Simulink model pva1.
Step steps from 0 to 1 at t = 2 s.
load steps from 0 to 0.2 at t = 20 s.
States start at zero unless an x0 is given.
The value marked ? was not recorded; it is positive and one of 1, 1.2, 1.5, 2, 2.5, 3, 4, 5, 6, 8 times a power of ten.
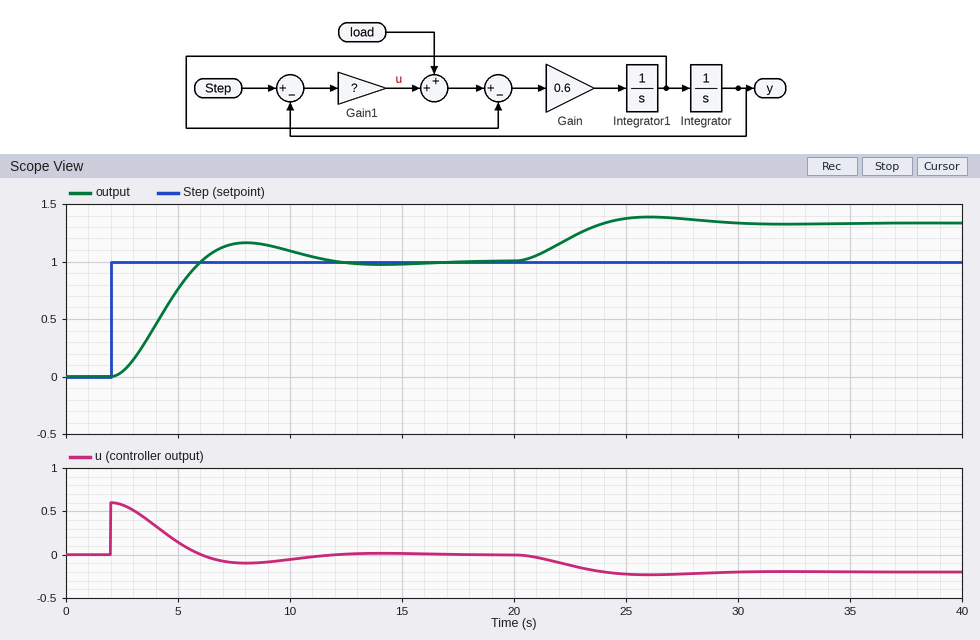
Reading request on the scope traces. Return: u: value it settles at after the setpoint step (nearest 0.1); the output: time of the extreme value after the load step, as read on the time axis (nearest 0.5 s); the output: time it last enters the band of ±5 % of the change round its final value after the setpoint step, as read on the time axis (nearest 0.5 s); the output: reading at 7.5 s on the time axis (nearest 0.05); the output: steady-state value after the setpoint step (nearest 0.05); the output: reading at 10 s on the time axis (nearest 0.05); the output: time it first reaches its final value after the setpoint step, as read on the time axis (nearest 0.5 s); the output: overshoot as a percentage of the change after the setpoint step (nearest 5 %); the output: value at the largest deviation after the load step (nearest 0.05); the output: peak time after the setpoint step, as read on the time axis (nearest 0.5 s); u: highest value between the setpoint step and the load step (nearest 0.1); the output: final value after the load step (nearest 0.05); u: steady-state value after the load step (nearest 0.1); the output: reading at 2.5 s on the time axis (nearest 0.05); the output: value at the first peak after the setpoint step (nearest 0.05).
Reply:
0.0
26.0 s
11.0 s
1.15
1.00
1.10
6.0 s
15 %
1.40
8.0 s
0.6
1.35
-0.2
0.05
1.15
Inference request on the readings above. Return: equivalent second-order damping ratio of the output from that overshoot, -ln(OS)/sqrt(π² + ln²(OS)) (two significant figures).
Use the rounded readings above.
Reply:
0.52
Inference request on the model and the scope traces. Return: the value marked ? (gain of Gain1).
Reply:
0.6
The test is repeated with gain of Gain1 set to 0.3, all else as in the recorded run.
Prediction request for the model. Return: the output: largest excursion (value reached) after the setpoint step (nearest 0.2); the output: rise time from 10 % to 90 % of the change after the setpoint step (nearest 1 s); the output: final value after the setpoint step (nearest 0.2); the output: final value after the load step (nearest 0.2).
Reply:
1.0
5 s
1.0
1.6
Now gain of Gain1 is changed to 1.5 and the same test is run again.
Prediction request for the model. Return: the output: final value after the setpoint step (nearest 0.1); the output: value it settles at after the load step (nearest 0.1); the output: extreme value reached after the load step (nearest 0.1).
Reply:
1.0
1.1
1.2
